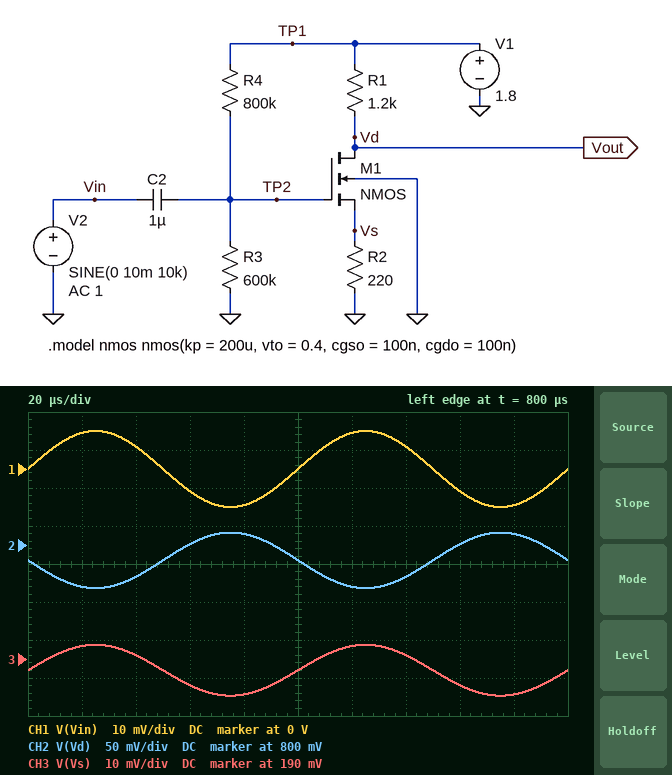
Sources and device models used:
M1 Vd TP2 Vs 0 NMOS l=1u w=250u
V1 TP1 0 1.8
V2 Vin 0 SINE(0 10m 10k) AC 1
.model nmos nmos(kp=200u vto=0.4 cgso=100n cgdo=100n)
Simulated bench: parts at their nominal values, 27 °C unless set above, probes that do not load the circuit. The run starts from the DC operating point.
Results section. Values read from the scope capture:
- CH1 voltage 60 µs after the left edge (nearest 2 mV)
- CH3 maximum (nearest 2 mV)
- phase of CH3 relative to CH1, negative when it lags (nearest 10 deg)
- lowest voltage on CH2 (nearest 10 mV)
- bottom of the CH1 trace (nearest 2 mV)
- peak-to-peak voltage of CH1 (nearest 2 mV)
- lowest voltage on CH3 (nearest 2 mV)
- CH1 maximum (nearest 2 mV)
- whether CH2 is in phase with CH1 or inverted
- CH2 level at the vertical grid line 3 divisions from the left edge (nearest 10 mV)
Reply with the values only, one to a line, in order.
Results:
-6 mV
194 mV
0 deg
740 mV
-10 mV
20 mV
180 mV
10 mV
inverted
800 mV
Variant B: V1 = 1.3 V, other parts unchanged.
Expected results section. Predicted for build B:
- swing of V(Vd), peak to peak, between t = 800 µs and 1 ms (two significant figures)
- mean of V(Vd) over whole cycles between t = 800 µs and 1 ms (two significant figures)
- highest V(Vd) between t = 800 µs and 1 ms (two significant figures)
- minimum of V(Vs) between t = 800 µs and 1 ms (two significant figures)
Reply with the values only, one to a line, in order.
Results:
57 mV
990 mV
1.0 V
51 mV
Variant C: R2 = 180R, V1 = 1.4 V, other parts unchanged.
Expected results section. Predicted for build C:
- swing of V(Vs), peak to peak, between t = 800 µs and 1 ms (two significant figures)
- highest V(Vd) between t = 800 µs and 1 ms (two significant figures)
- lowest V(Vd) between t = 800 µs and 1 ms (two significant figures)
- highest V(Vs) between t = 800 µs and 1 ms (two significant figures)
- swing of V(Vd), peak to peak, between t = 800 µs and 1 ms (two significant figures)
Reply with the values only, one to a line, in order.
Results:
11 mV
950 mV
880 mV
78 mV
71 mV
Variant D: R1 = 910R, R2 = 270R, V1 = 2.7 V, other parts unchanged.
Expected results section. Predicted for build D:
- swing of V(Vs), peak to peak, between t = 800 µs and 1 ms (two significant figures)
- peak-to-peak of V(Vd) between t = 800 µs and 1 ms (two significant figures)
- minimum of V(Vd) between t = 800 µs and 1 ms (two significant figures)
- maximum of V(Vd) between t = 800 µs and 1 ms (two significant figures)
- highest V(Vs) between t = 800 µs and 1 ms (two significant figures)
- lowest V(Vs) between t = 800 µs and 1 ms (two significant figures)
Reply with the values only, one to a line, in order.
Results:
16 mV
53 mV
1.0 V
1.1 V
500 mV
480 mV
